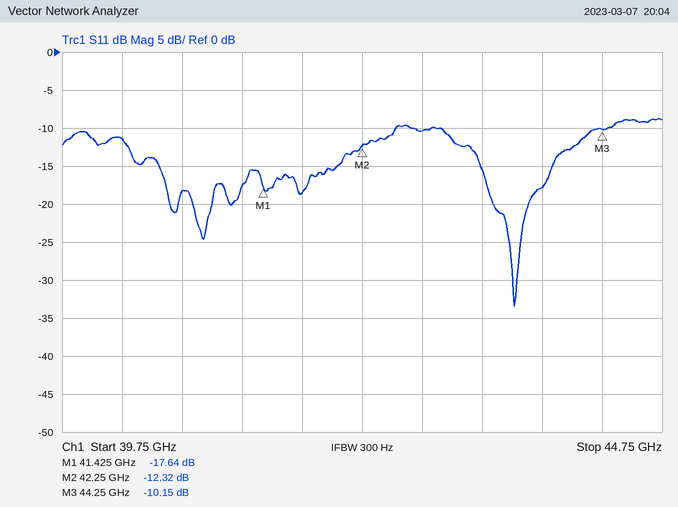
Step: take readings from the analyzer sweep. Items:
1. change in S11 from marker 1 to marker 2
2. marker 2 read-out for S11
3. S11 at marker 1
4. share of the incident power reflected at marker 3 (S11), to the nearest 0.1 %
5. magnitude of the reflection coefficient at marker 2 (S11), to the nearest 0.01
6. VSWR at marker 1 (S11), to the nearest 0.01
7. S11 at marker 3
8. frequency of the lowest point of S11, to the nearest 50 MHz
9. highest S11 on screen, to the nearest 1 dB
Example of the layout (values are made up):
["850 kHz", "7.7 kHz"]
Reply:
["5.32 dB", "-12.32 dB", "-17.64 dB", "9.7 %", "0.24", "1.30", "-10.15 dB", "43.50 GHz", "-9 dB"]
